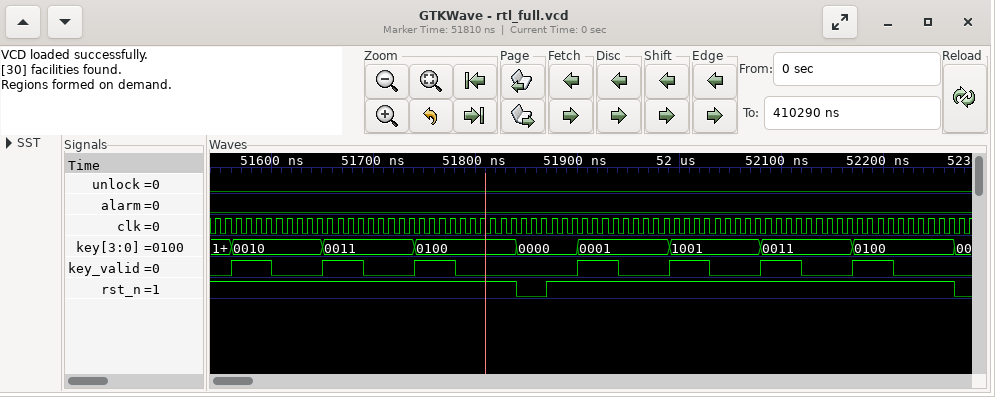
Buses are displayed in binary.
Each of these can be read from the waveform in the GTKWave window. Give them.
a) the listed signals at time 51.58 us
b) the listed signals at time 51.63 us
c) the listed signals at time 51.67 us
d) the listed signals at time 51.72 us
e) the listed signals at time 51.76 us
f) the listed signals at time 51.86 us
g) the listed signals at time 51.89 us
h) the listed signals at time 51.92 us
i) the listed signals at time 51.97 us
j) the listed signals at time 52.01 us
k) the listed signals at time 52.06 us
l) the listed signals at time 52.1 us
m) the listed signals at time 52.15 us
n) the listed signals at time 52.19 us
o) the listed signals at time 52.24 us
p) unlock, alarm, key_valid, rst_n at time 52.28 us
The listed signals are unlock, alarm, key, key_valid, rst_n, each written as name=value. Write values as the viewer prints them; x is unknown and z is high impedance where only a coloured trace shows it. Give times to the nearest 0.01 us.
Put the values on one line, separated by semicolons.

unlock=0, alarm=0, key=0010, key_valid=1, rst_n=1; unlock=0, alarm=0, key=0010, key_valid=0, rst_n=1; unlock=0, alarm=0, key=0011, key_valid=1, rst_n=1; unlock=0, alarm=0, key=0011, key_valid=0, rst_n=1; unlock=0, alarm=0, key=0100, key_valid=1, rst_n=1; unlock=0, alarm=0, key=0000, key_valid=0, rst_n=0; unlock=0, alarm=0, key=0000, key_valid=0, rst_n=1; unlock=0, alarm=0, key=0001, key_valid=1, rst_n=1; unlock=0, alarm=0, key=0001, key_valid=0, rst_n=1; unlock=0, alarm=0, key=1001, key_valid=1, rst_n=1; unlock=0, alarm=0, key=1001, key_valid=0, rst_n=1; unlock=0, alarm=0, key=0011, key_valid=1, rst_n=1; unlock=0, alarm=0, key=0011, key_valid=0, rst_n=1; unlock=0, alarm=0, key=0100, key_valid=1, rst_n=1; unlock=0, alarm=0, key=0100, key_valid=0, rst_n=1; unlock=0, alarm=0, key_valid=0, rst_n=0
